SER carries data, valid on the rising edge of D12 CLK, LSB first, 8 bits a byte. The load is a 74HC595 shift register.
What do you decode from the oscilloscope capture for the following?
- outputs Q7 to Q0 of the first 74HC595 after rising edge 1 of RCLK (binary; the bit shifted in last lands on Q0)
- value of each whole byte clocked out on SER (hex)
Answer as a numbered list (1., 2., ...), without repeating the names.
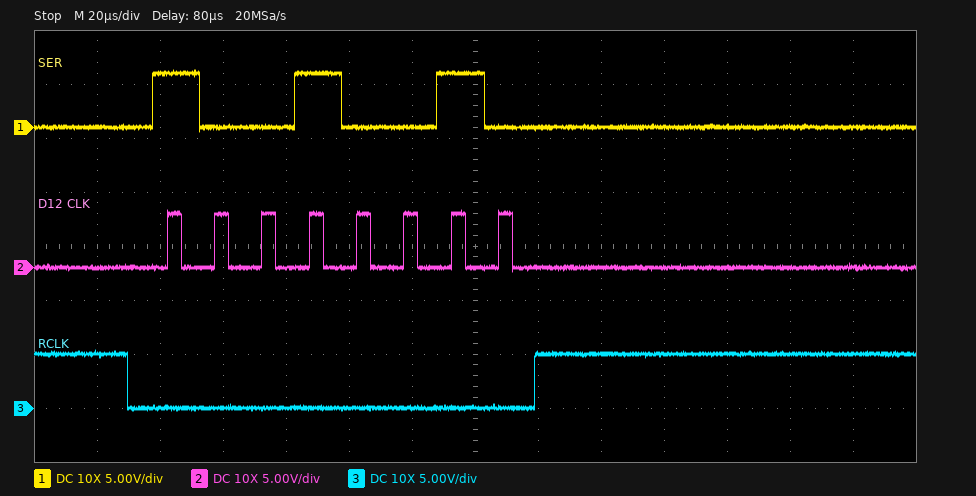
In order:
1. 10010010
2. 49
